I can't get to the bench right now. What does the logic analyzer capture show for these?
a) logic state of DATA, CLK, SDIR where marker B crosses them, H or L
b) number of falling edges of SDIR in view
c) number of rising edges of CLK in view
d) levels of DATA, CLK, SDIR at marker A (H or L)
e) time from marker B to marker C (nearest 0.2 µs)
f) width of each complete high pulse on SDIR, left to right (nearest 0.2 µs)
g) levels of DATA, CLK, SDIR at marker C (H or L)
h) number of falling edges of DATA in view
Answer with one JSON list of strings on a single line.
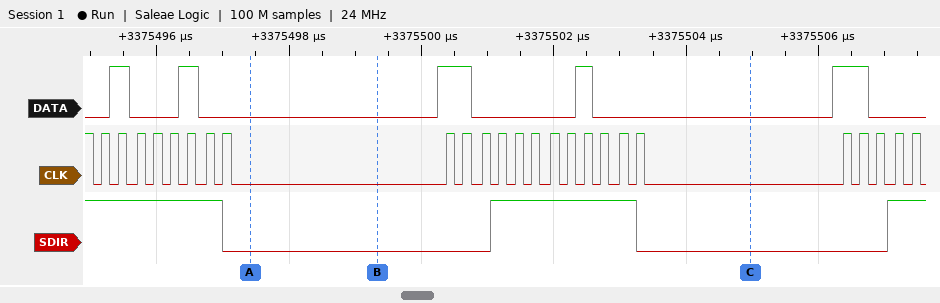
["DATA=L, CLK=L, SDIR=L", "2", "25", "DATA=L, CLK=L, SDIR=L", "5.6 µs", "2.2 µs", "DATA=L, CLK=L, SDIR=L", "5"]
